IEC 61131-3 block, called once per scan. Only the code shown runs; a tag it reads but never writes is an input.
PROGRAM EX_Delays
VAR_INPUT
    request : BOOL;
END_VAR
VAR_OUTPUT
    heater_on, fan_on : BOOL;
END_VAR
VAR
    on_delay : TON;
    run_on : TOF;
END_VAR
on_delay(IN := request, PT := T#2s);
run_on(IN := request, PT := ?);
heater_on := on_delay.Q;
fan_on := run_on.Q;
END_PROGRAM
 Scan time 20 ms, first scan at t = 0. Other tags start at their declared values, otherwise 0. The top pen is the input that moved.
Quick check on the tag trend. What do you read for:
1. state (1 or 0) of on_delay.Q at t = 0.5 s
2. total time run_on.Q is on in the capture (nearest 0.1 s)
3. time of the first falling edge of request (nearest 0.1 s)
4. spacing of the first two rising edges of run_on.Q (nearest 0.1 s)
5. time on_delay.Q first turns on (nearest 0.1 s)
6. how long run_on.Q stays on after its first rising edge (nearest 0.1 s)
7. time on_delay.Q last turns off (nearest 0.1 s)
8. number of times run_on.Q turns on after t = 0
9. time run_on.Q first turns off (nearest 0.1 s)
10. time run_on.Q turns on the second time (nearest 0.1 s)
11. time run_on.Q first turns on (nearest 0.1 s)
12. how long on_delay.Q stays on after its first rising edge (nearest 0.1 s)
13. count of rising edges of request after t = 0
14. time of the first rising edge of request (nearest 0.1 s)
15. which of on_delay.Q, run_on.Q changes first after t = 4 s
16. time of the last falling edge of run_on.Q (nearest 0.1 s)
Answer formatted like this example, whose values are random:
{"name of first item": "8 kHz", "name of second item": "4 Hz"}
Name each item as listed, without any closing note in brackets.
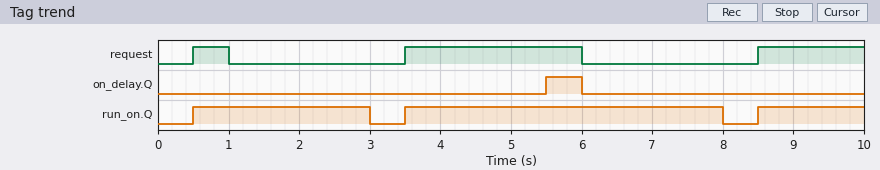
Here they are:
{"state (1 or 0) of on_delay.Q at t = 0.5 s": "0", "total time run_on.Q is on in the capture": "8.5 s", "time of the first falling edge of request": "1.0 s", "spacing of the first two rising edges of run_on.Q": "3.0 s", "time on_delay.Q first turns on": "5.5 s", "how long run_on.Q stays on after its first rising edge": "2.5 s", "time on_delay.Q last turns off": "6.0 s", "number of times run_on.Q turns on after t = 0": "3", "time run_on.Q first turns off": "3.0 s", "time run_on.Q turns on the second time": "3.5 s", "time run_on.Q first turns on": "0.5 s", "how long on_delay.Q stays on after its first rising edge": "0.5 s", "count of rising edges of request after t = 0": "3", "time of the first rising edge of request": "0.5 s", "which of on_delay.Q, run_on.Q changes first after t = 4 s": "on_delay.Q", "time of the last falling edge of run_on.Q": "8.0 s"}
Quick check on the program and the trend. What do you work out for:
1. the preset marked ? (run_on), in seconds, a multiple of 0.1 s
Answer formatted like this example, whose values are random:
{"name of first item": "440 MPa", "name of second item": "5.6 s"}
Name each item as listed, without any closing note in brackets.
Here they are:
{"the preset marked ? (run_on), in seconds, a multiple of 0.1 s": "2.0 s"}
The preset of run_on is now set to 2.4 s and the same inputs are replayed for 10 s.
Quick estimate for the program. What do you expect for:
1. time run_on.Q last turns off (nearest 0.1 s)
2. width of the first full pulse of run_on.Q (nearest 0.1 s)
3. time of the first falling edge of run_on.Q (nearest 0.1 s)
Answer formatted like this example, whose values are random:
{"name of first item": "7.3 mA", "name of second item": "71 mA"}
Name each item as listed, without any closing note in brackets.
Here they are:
{"time run_on.Q last turns off": "8.4 s", "width of the first full pulse of run_on.Q": "2.9 s", "time of the first falling edge of run_on.Q": "3.4 s"}
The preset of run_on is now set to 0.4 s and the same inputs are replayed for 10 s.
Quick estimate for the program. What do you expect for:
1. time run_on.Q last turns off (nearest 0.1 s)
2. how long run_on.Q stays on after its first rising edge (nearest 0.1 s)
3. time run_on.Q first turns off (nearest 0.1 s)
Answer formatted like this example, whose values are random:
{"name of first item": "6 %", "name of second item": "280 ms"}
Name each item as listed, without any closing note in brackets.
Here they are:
{"time run_on.Q last turns off": "6.4 s", "how long run_on.Q stays on after its first rising edge": "0.9 s", "time run_on.Q first turns off": "1.4 s"}
